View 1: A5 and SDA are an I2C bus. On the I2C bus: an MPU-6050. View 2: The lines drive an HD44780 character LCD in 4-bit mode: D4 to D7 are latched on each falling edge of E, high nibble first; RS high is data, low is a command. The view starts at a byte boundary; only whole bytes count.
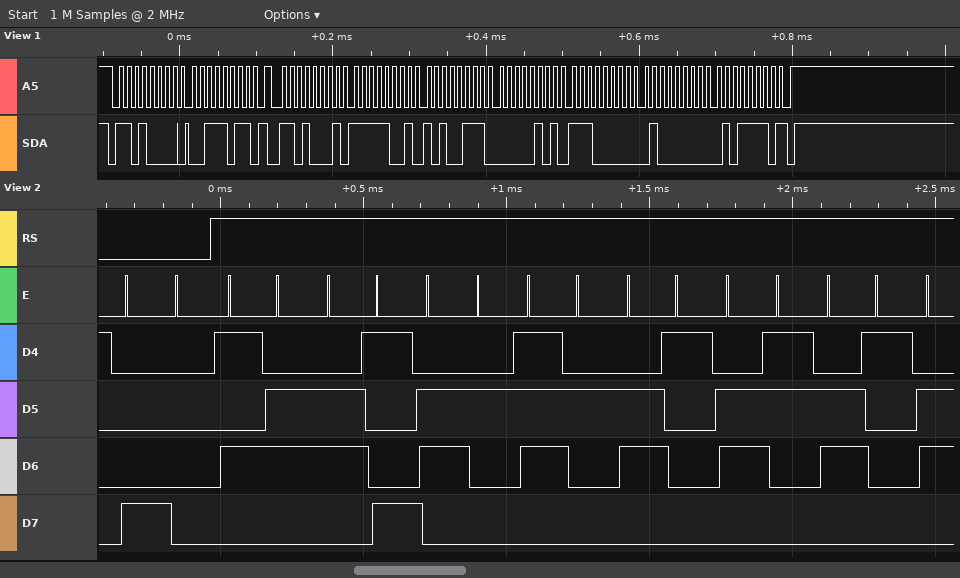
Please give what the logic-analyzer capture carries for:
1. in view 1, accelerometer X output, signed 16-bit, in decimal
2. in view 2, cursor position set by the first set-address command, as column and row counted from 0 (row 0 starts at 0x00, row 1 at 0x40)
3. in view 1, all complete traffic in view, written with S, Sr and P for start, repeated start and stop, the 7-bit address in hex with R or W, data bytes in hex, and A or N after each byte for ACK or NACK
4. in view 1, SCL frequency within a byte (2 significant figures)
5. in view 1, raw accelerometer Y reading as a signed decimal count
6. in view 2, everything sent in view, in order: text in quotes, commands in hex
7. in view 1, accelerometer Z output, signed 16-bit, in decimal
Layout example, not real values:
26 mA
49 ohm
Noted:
-1625
column 0, row 0
S 68W A 3B A Sr 68R A F9 A A7 A 05 A E0 A 40 A 5E N P
100 kHz
1504
0x80 "Vibraca"
16478
